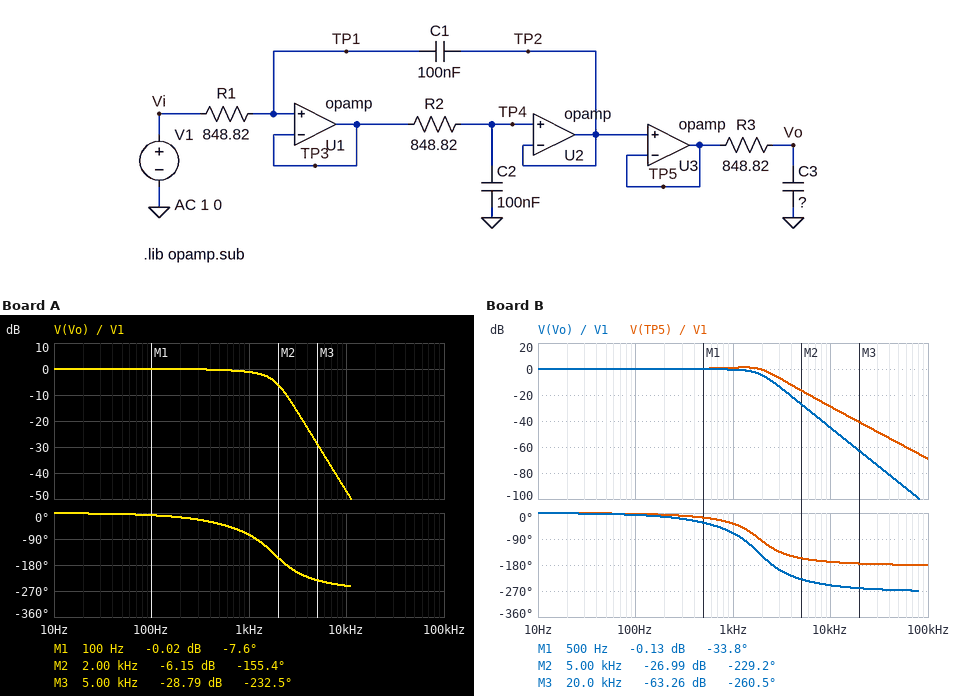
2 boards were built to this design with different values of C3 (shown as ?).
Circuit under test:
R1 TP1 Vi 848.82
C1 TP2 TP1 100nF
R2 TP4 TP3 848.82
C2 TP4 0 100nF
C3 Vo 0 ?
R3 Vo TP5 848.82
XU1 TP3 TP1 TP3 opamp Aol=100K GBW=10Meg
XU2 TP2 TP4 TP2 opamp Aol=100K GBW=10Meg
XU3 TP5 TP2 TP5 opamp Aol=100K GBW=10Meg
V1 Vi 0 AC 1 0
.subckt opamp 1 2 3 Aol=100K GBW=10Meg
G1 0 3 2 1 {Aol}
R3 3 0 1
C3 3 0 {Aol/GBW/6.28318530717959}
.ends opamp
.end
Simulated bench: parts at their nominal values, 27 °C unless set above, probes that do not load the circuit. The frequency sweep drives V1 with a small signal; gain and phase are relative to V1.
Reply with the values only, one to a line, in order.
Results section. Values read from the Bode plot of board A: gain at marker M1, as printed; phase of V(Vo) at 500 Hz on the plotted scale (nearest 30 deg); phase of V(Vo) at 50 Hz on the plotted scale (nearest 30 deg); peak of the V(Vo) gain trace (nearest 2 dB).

-0.02 dB
-30 deg
0 deg
0 dB
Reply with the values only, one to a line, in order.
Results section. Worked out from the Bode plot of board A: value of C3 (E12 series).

150 nF
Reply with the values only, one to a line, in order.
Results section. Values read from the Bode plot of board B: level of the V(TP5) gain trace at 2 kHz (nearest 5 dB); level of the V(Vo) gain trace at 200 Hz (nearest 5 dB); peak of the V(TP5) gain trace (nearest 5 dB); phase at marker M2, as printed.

0 dB
0 dB
0 dB
-229.2 deg
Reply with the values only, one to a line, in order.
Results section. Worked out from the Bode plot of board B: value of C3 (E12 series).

120 nF
